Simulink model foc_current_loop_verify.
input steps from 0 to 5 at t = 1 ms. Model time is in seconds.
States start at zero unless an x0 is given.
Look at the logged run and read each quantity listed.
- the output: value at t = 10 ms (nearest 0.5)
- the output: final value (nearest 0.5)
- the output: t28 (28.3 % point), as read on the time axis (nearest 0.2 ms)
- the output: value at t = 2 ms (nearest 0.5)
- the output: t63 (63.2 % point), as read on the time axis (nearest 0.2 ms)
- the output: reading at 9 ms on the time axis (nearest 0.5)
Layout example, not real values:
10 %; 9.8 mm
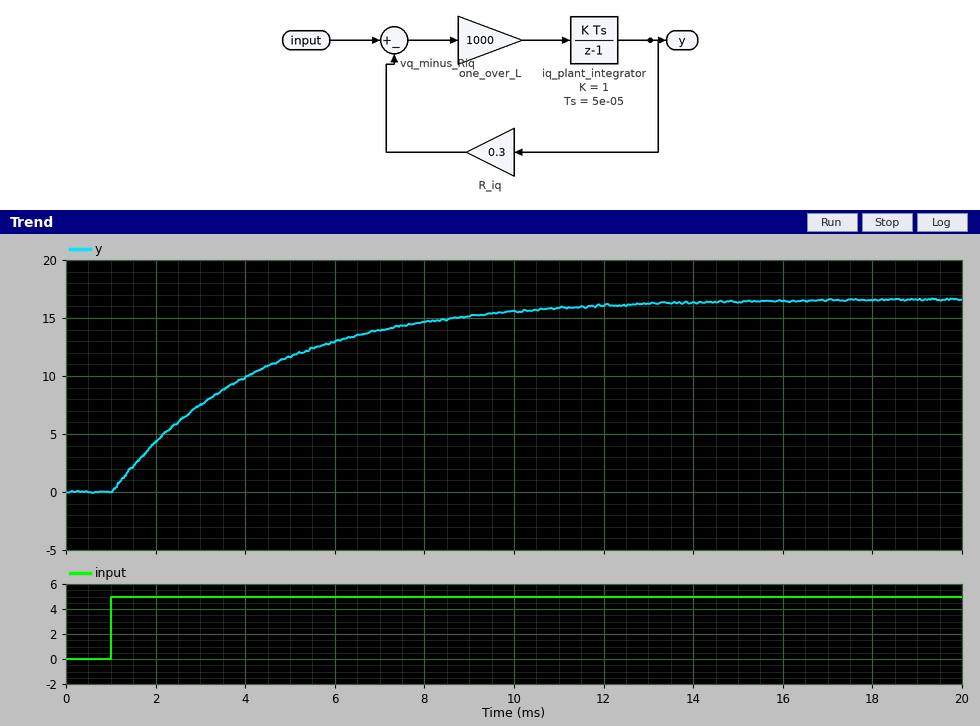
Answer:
15.5; 16.5; 2.2 ms; 4.5; 4.4 ms; 15.0
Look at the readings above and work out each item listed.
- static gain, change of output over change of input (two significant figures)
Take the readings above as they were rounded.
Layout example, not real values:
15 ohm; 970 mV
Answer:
3.3
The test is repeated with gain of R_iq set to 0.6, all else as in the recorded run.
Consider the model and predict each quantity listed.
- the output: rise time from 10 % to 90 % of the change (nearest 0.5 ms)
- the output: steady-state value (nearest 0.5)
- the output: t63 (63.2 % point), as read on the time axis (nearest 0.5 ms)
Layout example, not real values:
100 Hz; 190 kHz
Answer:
3.5 ms; 8.5; 2.5 ms
